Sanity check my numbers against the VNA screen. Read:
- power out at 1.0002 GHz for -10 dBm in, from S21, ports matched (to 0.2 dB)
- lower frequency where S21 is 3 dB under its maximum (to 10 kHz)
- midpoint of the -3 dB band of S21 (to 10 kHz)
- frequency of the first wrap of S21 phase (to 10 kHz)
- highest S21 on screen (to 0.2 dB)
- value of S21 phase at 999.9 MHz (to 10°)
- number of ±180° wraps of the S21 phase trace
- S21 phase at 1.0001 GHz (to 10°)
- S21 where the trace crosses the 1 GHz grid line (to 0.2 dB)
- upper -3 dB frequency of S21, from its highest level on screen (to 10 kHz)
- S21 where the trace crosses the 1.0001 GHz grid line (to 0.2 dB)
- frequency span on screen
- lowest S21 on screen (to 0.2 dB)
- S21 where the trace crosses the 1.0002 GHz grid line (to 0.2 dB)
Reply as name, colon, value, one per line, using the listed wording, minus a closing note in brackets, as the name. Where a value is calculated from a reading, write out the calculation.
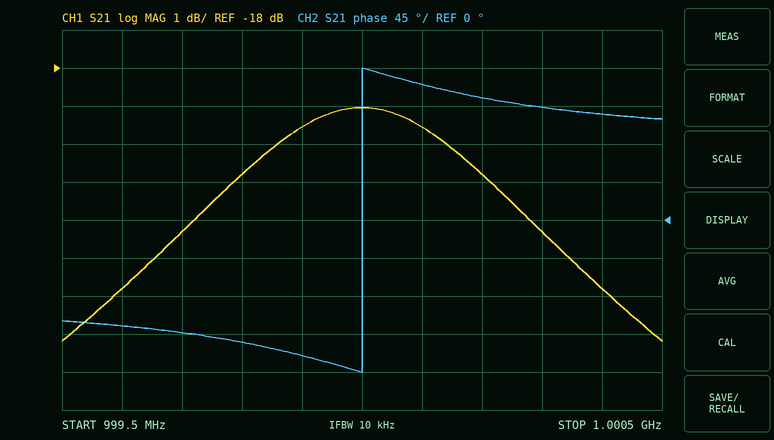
power out at 1.0002 GHz for -10 dBm in, from S21, ports matched: -10 dBm + (-20.8 dB) = -30.8 dBm
lower frequency where S21 is 3 dB under its maximum: 999.72 MHz
midpoint of the -3 dB band of S21: 1.00000 GHz
frequency of the first wrap of S21 phase: 1.00000 GHz
highest S21 on screen: -19.0 dB
value of S21 phase at 999.9 MHz: -160°
number of ±180° wraps of the S21 phase trace: 1
S21 phase at 1.0001 GHz: 160°
S21 where the trace crosses the 1 GHz grid line: -19.0 dB
upper -3 dB frequency of S21, from its highest level on screen: 1.00028 GHz
S21 where the trace crosses the 1.0001 GHz grid line: -19.6 dB
frequency span on screen: 1 MHz
lowest S21 on screen: -25.2 dB
S21 where the trace crosses the 1.0002 GHz grid line: -20.8 dB
